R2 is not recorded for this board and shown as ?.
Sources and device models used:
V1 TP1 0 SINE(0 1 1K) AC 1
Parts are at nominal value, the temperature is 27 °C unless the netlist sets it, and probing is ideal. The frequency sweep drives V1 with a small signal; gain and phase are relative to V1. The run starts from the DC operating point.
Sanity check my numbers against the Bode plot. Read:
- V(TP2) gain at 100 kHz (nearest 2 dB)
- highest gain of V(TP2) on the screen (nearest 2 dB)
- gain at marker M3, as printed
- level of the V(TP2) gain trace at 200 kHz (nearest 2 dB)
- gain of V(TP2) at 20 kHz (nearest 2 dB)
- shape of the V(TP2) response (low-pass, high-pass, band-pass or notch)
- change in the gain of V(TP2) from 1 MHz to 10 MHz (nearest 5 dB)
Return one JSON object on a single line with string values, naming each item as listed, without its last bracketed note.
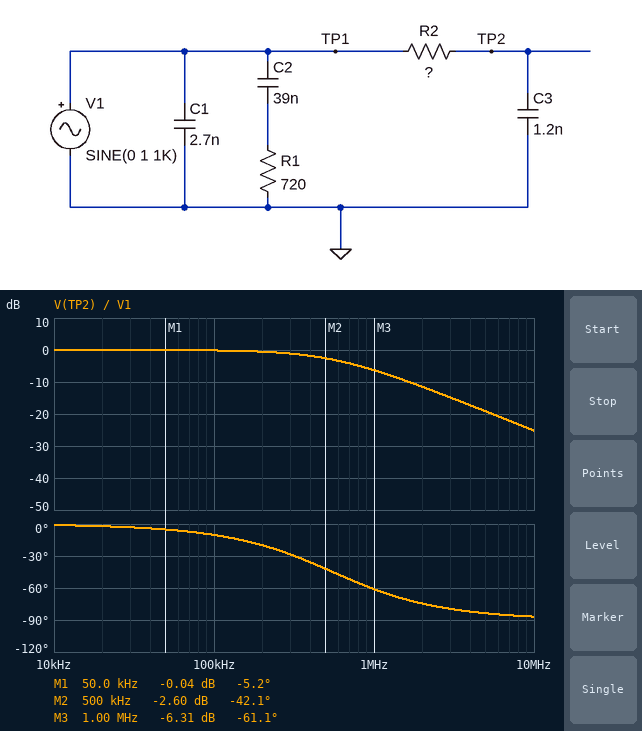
{"V(TP2) gain at 100 kHz": "0 dB", "highest gain of V(TP2) on the screen": "0 dB", "gain at marker M3, as printed": "-6.31 dB", "level of the V(TP2) gain trace at 200 kHz": "0 dB", "gain of V(TP2) at 20 kHz": "0 dB", "shape of the V(TP2) response": "low-pass", "change in the gain of V(TP2) from 1 MHz to 10 MHz": "-20 dB"}
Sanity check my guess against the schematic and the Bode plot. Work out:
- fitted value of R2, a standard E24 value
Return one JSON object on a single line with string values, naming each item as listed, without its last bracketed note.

{"fitted value of R2, a standard E24 value": "240 Ω"}
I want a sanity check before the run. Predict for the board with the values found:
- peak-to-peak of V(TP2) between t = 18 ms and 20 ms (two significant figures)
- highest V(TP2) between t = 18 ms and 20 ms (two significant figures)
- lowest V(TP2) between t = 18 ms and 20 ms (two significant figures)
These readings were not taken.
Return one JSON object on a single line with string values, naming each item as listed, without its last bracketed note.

{"peak-to-peak of V(TP2) between t = 18 ms and 20 ms": "2.0 V", "highest V(TP2) between t = 18 ms and 20 ms": "1.0 V", "lowest V(TP2) between t = 18 ms and 20 ms": "-1.0 V"}
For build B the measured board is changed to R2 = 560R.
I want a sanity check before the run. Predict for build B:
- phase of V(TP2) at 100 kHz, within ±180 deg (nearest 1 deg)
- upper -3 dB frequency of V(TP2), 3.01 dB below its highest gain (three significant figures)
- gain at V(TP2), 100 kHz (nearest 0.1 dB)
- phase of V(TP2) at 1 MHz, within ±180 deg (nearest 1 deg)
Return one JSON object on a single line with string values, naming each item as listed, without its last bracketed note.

{"phase of V(TP2) at 100 kHz, within ±180 deg": "-23 deg", "upper -3 dB frequency of V(TP2), 3.01 dB below its highest gain": "237 kHz", "gain at V(TP2), 100 kHz": "-0.7 dB", "phase of V(TP2) at 1 MHz, within ±180 deg": "-77 deg"}
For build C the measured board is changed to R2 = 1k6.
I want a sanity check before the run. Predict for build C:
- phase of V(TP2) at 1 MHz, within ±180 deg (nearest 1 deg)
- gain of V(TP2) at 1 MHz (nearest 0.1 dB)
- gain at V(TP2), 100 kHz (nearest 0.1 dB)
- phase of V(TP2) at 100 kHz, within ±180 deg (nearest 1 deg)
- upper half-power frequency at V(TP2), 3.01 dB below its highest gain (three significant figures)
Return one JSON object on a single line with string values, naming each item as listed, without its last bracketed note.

{"phase of V(TP2) at 1 MHz, within ±180 deg": "-85 deg", "gain of V(TP2) at 1 MHz": "-21.7 dB", "gain at V(TP2), 100 kHz": "-3.9 dB", "phase of V(TP2) at 100 kHz, within ±180 deg": "-50 deg", "upper half-power frequency at V(TP2), 3.01 dB below its highest gain": "82.9 kHz"}
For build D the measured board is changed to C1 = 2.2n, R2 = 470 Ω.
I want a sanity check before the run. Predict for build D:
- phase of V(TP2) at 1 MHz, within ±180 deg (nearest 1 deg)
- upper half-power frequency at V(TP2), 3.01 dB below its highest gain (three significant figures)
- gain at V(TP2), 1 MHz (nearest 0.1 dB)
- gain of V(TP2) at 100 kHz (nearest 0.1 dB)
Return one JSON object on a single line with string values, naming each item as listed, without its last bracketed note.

{"phase of V(TP2) at 1 MHz, within ±180 deg": "-74 deg", "upper half-power frequency at V(TP2), 3.01 dB below its highest gain": "282 kHz", "gain at V(TP2), 1 MHz": "-11.3 dB", "gain of V(TP2) at 100 kHz": "-0.5 dB"}
